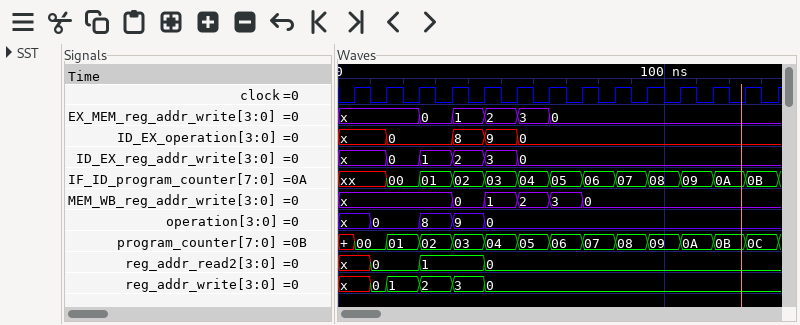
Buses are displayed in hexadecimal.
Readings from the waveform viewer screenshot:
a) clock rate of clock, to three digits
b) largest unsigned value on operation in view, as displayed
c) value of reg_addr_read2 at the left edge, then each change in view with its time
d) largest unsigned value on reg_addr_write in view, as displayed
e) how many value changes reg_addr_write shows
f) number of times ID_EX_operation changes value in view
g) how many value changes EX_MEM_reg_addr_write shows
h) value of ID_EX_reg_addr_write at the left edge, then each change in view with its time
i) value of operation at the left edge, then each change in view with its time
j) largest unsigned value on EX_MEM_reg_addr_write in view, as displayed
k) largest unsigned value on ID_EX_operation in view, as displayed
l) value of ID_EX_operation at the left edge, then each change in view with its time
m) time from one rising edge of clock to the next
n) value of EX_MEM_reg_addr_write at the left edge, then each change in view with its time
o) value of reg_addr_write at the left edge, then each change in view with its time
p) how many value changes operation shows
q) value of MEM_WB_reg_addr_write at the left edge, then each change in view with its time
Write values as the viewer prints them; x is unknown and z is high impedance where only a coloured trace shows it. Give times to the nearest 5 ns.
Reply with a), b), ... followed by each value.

a) 100 MHz
b) 9
c) x, 0 at 10 ns, 1 at 25 ns, 0 at 45 ns
d) 3
e) 5
f) 4
g) 5
h) x, 0 at 15 ns, 1 at 25 ns, 2 at 35 ns, 3 at 45 ns, 0 at 55 ns
i) x, 0 at 10 ns, 8 at 25 ns, 9 at 35 ns, 0 at 45 ns
j) 3
k) 9
l) x, 0 at 15 ns, 8 at 35 ns, 9 at 45 ns, 0 at 55 ns
m) 10 ns
n) x, 0 at 25 ns, 1 at 35 ns, 2 at 45 ns, 3 at 55 ns, 0 at 65 ns
o) x, 0 at 10 ns, 1 at 15 ns, 2 at 25 ns, 3 at 35 ns, 0 at 45 ns
p) 4
q) x, 0 at 35 ns, 1 at 45 ns, 2 at 55 ns, 3 at 65 ns, 0 at 75 ns
